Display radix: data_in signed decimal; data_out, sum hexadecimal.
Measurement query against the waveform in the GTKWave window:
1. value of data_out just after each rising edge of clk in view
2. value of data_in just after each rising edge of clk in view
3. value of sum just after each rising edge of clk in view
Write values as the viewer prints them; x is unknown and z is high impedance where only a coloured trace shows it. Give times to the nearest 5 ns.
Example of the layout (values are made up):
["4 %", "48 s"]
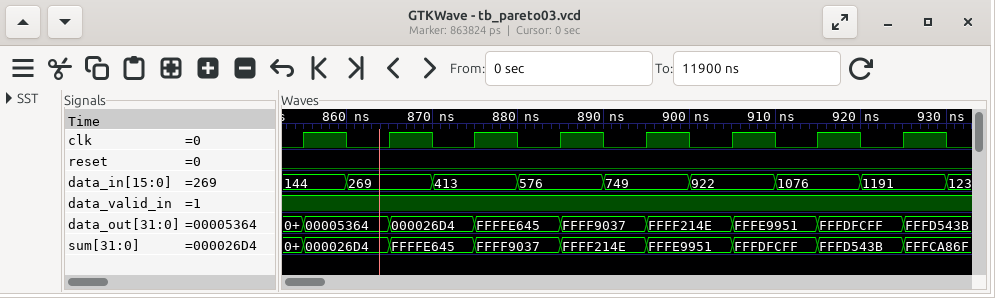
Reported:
["00005364, 000026D4, FFFFE645, FFFF9037, FFFF214E, FFFE9951, FFFDFCFF, FFFD543B", "144, 269, 413, 576, 749, 922, 1076, 1191", "000026D4, FFFFE645, FFFF9037, FFFF214E, FFFE9951, FFFDFCFF, FFFD543B, FFFCA86F"]
